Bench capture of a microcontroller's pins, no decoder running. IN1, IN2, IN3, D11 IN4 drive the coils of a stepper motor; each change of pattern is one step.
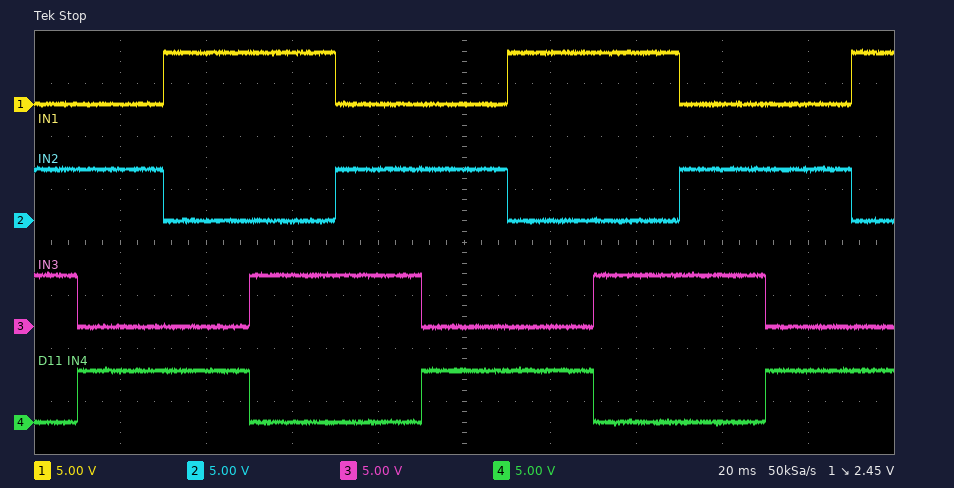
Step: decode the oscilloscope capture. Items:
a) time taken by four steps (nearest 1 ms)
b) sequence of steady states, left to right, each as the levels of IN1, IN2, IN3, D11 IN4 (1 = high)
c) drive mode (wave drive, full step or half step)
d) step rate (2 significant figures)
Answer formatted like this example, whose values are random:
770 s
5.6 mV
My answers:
80 ms
0110 0101 1001 1010 0110 0101 1001 1010 0110 0101 1001
full step
50 steps/s
